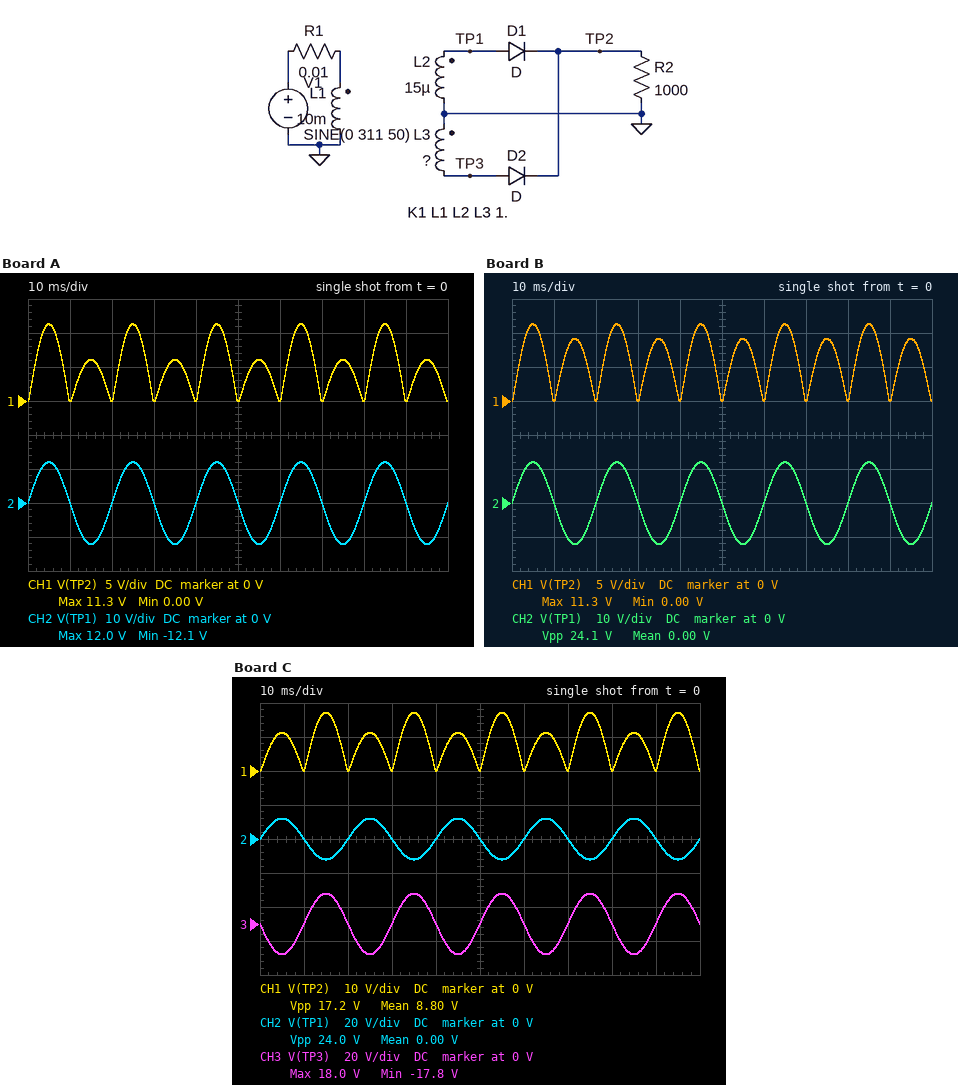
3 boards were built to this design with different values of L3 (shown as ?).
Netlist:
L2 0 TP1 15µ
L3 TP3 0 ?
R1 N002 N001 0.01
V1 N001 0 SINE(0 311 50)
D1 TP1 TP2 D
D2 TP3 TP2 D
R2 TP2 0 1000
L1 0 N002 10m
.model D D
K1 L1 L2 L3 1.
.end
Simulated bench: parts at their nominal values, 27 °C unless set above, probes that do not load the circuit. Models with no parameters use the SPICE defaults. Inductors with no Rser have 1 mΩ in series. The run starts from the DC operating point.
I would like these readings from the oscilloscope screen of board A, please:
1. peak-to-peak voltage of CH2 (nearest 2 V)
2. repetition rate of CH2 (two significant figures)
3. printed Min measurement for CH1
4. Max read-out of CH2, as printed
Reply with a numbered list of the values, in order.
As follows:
1. 24 V
2. 50 Hz
3. 0.00 V
4. 12.0 V
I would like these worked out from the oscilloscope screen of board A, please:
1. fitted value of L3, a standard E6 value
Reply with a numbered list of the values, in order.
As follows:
1. 4.7 µH
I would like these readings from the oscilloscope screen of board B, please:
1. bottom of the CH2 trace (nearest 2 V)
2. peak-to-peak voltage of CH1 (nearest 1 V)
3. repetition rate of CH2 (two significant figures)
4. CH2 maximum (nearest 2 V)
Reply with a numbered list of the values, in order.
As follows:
1. -12 V
2. 11 V
3. 50 Hz
4. 12 V
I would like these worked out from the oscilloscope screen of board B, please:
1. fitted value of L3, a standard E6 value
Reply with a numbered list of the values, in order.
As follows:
1. 10 µH
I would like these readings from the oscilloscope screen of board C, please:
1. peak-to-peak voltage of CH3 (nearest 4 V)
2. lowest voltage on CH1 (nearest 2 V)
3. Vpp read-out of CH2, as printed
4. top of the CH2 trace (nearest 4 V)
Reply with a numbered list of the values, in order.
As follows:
1. 36 V
2. 0 V
3. 24.0 V
4. 12 V
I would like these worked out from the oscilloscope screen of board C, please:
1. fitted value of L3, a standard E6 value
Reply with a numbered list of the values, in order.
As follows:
1. 33 µH
